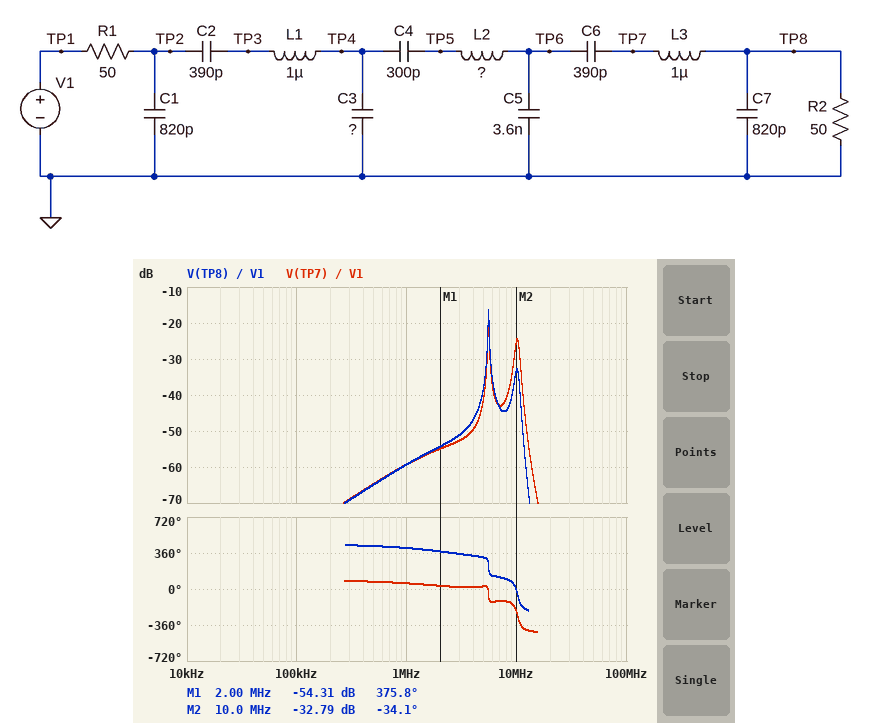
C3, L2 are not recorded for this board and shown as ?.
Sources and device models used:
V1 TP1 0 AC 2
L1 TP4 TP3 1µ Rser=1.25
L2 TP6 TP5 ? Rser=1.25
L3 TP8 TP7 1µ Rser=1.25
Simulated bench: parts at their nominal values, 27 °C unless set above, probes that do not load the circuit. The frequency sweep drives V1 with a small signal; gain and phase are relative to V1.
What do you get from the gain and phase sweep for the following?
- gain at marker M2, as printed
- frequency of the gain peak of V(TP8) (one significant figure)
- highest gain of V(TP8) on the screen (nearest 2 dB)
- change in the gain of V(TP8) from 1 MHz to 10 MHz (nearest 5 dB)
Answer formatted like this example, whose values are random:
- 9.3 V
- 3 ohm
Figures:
- -32.79 dB
- 6 MHz
- -16 dB
- 25 dB
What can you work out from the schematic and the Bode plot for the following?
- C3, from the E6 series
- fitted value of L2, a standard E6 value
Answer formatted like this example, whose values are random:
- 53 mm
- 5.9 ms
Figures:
- 2.2 nF
- 3.3 µH
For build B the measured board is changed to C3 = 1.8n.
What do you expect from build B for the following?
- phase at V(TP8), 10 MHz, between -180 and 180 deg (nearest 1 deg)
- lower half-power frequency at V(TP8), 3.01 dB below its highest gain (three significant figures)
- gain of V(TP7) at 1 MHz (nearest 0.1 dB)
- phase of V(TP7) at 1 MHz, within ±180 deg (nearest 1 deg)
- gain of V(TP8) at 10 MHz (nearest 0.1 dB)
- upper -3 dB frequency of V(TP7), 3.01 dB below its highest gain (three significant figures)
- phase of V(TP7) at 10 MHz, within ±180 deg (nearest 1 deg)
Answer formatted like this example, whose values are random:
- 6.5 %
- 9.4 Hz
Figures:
- -23 deg
- 5.51 MHz
- -57.9 dB
- 57 deg
- -31.7 dB
- 5.61 MHz
- 126 deg
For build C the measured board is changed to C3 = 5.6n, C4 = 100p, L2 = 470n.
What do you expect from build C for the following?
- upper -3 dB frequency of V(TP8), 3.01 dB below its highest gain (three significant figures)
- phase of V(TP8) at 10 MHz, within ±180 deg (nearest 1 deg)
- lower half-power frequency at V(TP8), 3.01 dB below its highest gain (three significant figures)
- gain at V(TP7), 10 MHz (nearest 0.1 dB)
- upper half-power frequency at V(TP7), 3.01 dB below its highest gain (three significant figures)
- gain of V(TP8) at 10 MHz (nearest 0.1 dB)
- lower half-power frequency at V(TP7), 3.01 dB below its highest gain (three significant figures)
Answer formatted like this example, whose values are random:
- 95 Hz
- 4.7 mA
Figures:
- 10.3 MHz
- 109 deg
- 9.44 MHz
- -32.3 dB
- 10.4 MHz
- -40.5 dB
- 9.52 MHz
